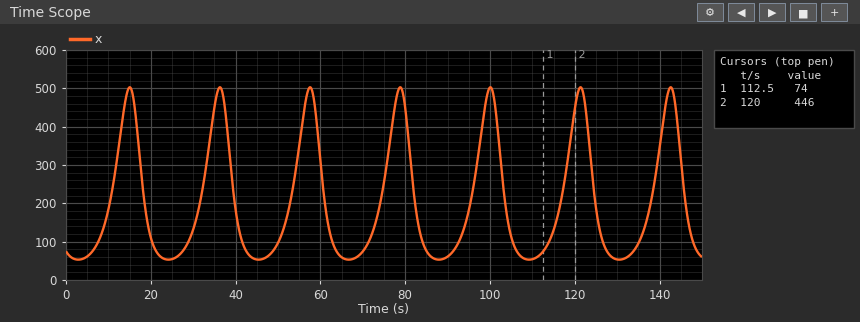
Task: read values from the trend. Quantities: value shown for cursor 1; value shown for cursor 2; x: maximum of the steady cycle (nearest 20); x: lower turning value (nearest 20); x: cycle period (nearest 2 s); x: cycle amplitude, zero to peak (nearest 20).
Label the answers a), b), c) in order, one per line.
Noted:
a) 74
b) 446
c) 500
d) 60
e) 22 s
f) 220
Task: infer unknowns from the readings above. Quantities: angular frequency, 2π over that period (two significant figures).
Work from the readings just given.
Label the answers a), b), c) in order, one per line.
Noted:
a) 0.29 rad/s
